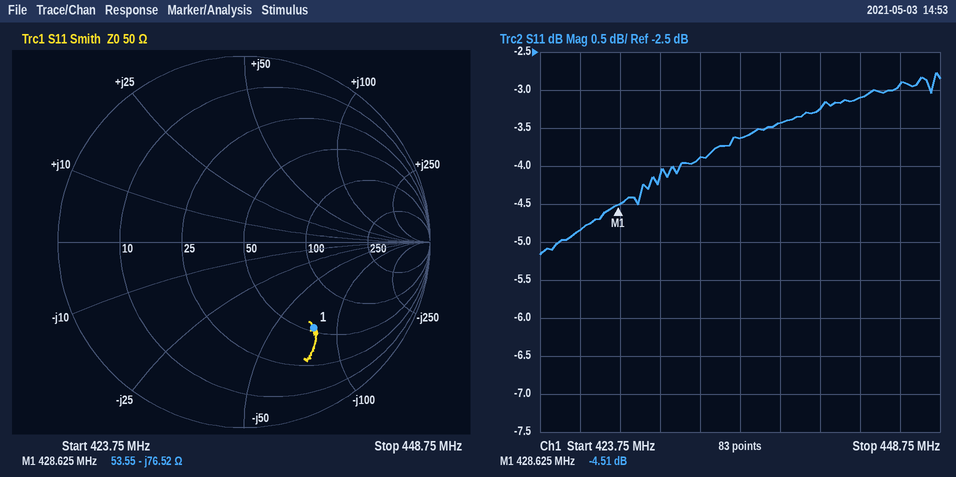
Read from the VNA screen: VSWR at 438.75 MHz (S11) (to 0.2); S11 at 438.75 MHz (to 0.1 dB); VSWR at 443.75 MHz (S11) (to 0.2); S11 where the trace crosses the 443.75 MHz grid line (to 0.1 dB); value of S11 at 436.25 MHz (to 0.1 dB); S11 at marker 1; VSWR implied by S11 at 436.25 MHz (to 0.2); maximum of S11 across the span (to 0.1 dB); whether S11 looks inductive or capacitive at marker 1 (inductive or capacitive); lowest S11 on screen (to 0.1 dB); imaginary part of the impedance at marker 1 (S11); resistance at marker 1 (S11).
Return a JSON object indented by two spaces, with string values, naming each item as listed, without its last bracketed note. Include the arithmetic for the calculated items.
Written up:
{
  "VSWR at 438.75 MHz (S11)": "|Γ| = 10^(-3.4/20) = 0.6761; VSWR = (1 + 0.6761)/(1 − 0.6761) ≈ 5.2",
  "S11 at 438.75 MHz": "-3.4 dB",
  "VSWR at 443.75 MHz (S11)": "|Γ| = 10^(-3.1/20) = 0.6998; VSWR = (1 + 0.6998)/(1 − 0.6998) ≈ 5.66, so 5.6 to the nearest 0.2",
  "S11 where the trace crosses the 443.75 MHz grid line": "-3.1 dB",
  "value of S11 at 436.25 MHz": "-3.6 dB",
  "S11 at marker 1": "-4.51 dB",
  "VSWR implied by S11 at 436.25 MHz": "|Γ| = 10^(-3.6/20) = 0.6607; VSWR = (1 + 0.6607)/(1 − 0.6607) ≈ 4.89, so 4.8 to the nearest 0.2",
  "maximum of S11 across the span": "-2.8 dB",
  "whether S11 looks inductive or capacitive at marker 1": "capacitive",
  "lowest S11 on screen": "-5.2 dB",
  "imaginary part of the impedance at marker 1": "-76.52 Ω",
  "resistance at marker 1": "53.55 Ω"
}
